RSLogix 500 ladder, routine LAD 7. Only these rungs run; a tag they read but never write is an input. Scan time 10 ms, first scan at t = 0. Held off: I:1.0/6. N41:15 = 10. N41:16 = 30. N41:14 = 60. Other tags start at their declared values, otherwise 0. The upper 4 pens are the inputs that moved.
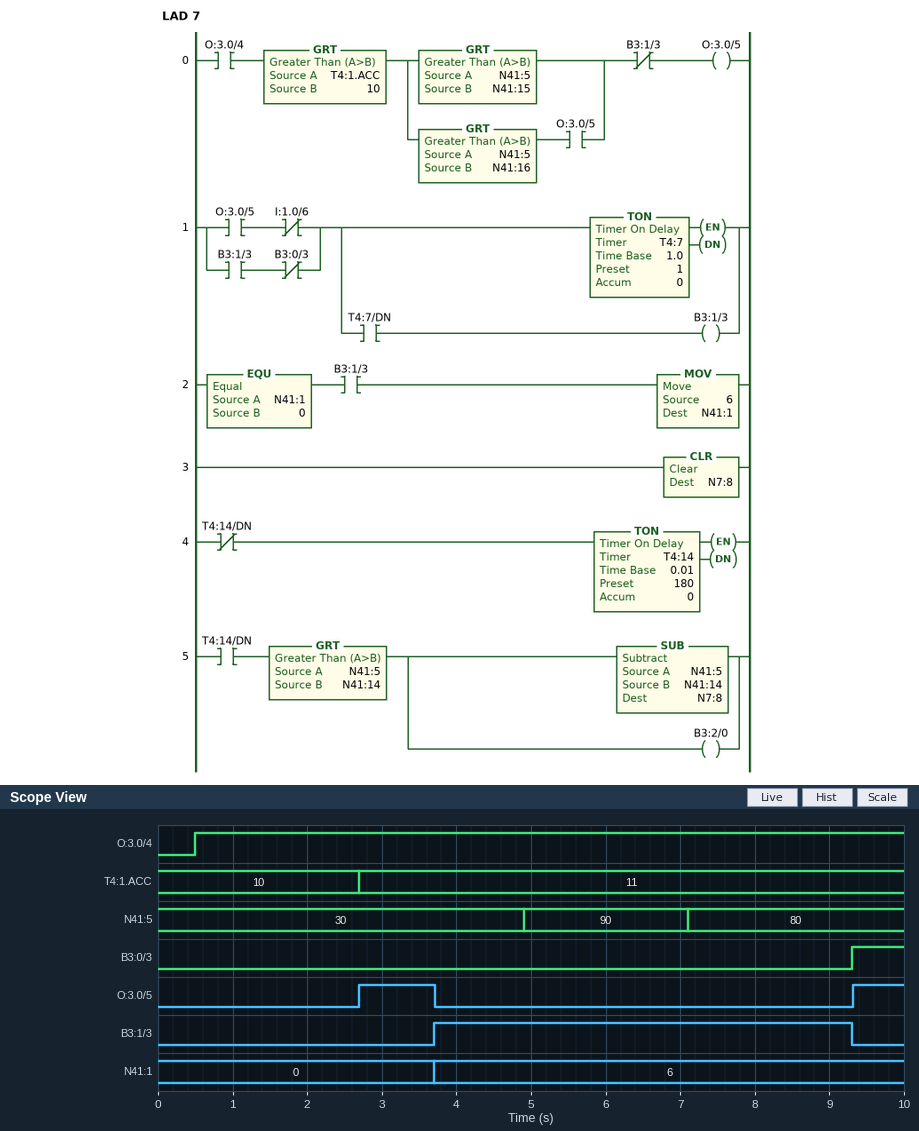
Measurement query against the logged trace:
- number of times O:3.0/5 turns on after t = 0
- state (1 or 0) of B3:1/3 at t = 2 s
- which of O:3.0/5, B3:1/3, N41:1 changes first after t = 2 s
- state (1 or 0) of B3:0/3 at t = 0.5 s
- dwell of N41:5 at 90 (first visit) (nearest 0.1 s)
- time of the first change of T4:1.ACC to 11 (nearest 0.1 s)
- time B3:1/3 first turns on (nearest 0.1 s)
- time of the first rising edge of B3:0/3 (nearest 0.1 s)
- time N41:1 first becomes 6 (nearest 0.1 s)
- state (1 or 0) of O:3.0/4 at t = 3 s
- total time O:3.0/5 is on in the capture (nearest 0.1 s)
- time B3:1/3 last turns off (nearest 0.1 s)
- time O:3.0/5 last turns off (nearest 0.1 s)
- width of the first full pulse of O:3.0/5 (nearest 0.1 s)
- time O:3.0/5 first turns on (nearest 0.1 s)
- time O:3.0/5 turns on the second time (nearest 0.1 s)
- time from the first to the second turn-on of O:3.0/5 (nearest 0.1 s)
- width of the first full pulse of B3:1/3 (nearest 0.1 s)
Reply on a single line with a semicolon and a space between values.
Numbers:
2; 0; O:3.0/5; 0; 2.2 s; 2.7 s; 3.7 s; 9.3 s; 3.7 s; 1; 1.7 s; 9.3 s; 3.7 s; 1.0 s; 2.7 s; 9.3 s; 6.6 s; 5.6 s
